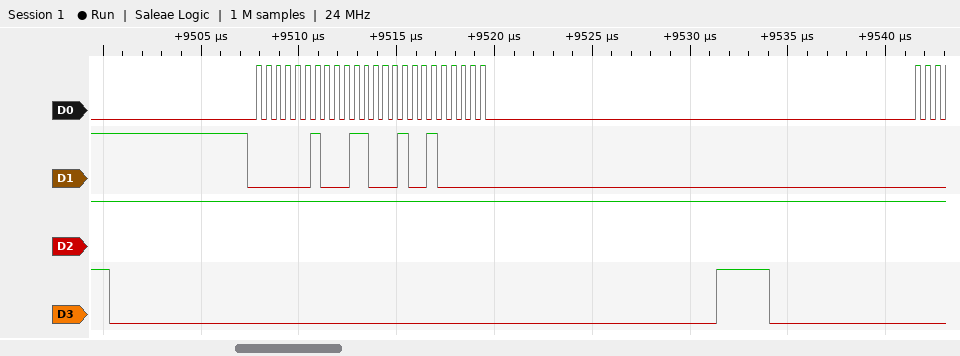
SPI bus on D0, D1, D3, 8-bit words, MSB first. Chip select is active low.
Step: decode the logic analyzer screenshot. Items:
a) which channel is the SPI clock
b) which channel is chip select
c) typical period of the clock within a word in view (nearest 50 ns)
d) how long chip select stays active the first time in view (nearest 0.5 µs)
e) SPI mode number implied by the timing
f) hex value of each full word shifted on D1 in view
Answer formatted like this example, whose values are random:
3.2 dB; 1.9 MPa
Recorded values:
D0; D3; 500 ns; 31 µs; 0; 02, 31, 20
